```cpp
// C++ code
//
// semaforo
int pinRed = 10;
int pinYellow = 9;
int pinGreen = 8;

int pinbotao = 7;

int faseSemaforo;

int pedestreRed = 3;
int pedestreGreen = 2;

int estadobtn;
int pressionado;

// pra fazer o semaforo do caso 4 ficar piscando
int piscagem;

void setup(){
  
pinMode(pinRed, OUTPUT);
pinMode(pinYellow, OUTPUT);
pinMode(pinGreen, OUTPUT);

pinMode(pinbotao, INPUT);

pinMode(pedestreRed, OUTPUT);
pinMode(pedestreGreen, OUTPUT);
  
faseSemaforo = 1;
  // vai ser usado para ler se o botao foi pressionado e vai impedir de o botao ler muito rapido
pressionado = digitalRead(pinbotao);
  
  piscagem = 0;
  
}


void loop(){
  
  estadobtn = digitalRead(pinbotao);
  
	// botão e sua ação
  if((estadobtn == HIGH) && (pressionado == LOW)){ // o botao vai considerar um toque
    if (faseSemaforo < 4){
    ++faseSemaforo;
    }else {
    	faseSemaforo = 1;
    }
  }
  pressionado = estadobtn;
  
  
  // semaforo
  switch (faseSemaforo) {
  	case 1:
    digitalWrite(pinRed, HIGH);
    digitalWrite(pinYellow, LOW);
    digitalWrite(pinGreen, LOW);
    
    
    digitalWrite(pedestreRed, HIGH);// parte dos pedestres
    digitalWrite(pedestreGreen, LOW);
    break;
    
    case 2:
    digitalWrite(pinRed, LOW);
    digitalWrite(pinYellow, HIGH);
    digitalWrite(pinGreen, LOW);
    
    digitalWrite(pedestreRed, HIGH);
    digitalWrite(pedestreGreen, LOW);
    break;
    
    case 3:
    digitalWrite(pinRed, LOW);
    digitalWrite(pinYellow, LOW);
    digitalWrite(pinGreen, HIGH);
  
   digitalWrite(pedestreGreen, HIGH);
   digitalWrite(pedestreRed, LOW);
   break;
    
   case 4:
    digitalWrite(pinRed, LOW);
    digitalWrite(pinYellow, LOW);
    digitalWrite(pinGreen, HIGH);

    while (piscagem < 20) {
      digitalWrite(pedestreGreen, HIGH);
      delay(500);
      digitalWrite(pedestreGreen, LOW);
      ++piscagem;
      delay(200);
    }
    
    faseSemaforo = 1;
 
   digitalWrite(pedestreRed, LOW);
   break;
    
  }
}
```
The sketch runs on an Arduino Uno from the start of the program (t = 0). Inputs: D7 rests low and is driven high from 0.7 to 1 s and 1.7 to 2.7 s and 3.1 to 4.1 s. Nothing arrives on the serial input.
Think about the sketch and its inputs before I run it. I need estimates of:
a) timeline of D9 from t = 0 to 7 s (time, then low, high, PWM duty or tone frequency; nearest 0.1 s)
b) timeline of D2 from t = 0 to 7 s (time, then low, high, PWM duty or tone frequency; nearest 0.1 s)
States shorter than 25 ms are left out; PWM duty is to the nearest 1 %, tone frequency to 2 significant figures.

0 s low; 0.7 s high; 1.7 s low
0 s low; 1.7 s high; 3.6 s low; 3.8 s high; 4.3 s low; 4.5 s high; 5 s low; 5.2 s high; 5.7 s low; 5.9 s high; 6.4 s low; 6.6 s high
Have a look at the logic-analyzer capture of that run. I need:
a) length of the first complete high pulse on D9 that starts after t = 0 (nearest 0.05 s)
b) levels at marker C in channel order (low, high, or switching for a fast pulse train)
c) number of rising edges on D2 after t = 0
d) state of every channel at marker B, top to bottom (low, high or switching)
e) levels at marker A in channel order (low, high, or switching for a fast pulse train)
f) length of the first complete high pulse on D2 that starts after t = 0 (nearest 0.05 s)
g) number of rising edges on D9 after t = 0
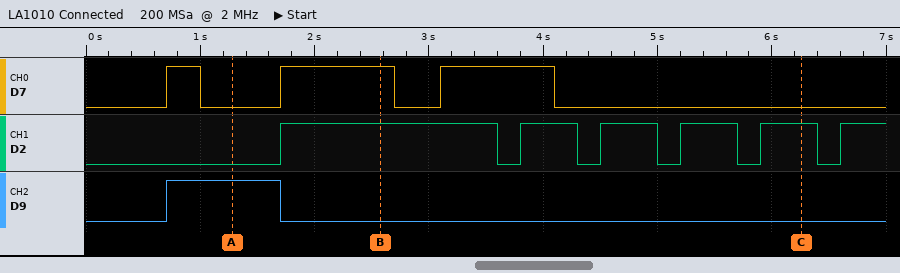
1.00 s
D7 low, D2 high, D9 low
6
D7 high, D2 high, D9 low
D7 low, D2 low, D9 high
1.90 s
1
